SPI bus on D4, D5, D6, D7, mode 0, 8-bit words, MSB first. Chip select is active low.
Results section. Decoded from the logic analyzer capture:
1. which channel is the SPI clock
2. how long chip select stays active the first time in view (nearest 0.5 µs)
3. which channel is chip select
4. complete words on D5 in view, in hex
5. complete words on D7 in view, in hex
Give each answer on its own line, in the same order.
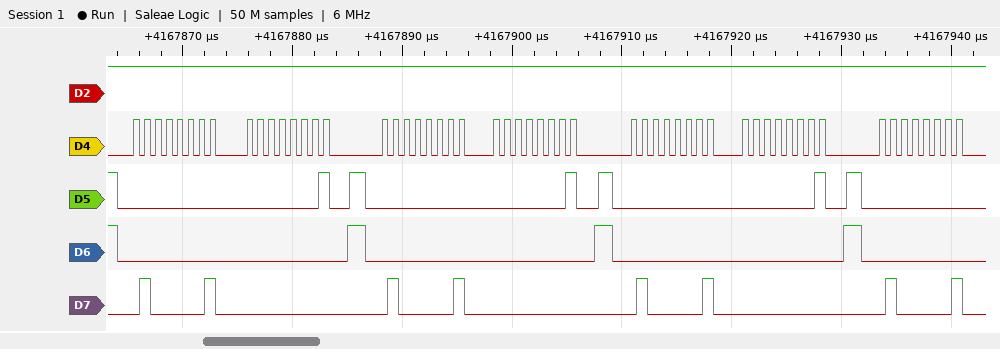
D4
21 µs
D6
00, 01, 00, 01, 00, 01, 00
41, 00, 41, 00, 41, 00, 41
